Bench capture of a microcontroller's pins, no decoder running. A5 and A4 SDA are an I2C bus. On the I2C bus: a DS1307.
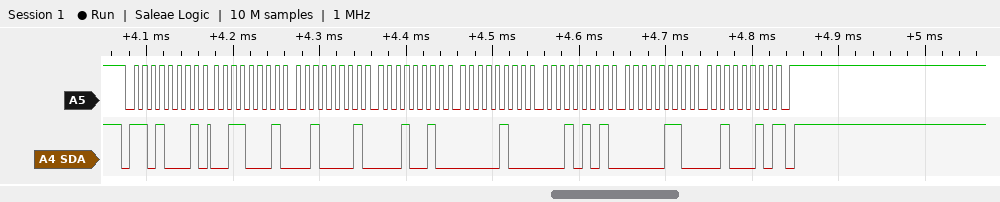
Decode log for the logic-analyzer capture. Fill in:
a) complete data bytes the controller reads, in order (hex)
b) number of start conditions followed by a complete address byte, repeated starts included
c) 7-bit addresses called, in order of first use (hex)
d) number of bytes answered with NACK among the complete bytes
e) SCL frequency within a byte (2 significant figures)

31 21 12 04 15 06 22
1
0x68
1
100 kHz
